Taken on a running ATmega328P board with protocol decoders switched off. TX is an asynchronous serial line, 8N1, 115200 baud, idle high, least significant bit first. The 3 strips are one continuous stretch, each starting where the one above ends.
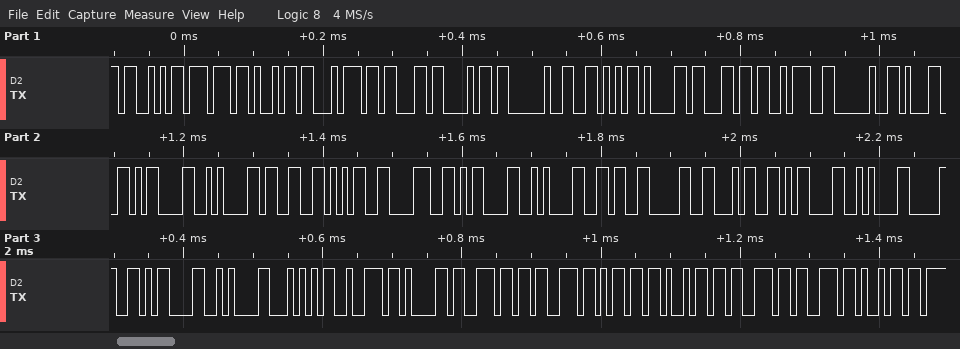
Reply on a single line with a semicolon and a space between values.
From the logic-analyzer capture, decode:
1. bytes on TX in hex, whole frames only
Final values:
53 77 69 74 63 68 20 56 61 6C 3A 20 31 0D 0A 33 35 38 0D 0A 36 30 34 0D 0A 30 0D 0A 54 72 61 6E 73 6D 69 73 73 69
